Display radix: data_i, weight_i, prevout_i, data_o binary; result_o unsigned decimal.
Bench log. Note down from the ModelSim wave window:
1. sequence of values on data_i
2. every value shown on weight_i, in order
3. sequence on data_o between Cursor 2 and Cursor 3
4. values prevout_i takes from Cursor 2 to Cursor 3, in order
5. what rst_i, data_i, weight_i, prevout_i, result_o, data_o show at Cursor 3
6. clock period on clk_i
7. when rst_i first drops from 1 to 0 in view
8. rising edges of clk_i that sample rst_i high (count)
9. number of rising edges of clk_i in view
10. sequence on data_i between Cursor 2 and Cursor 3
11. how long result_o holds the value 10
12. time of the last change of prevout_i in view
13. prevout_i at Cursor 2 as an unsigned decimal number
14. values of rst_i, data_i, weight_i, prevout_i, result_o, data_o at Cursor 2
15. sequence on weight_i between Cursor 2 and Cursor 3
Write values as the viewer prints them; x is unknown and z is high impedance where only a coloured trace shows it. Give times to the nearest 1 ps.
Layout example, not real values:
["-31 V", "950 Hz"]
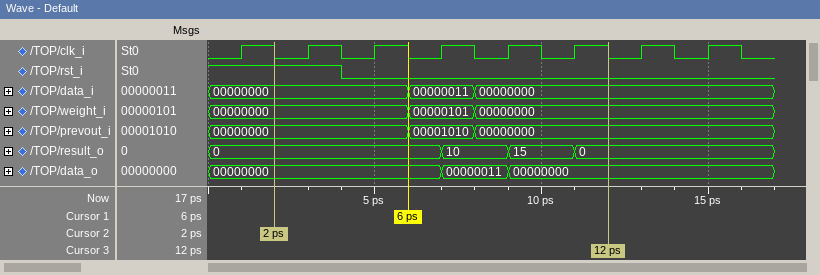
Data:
["00000000, 00000011, 00000000", "00000000, 00000101, 00000000", "00000000, 00000011, 00000000", "00000000, 00001010, 00000000", "rst_i=0, data_i=00000000, weight_i=00000000, prevout_i=00000000, result_o=0, data_o=00000000", "2 ps", "4 ps", "2", "8", "00000000, 00000011, 00000000", "2 ps", "8 ps", "0", "rst_i=1, data_i=00000000, weight_i=00000000, prevout_i=00000000, result_o=0, data_o=00000000", "00000000, 00000101, 00000000"]
